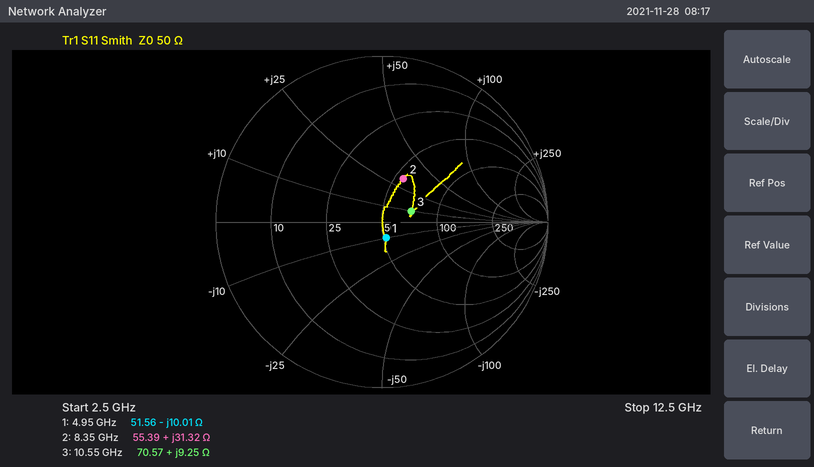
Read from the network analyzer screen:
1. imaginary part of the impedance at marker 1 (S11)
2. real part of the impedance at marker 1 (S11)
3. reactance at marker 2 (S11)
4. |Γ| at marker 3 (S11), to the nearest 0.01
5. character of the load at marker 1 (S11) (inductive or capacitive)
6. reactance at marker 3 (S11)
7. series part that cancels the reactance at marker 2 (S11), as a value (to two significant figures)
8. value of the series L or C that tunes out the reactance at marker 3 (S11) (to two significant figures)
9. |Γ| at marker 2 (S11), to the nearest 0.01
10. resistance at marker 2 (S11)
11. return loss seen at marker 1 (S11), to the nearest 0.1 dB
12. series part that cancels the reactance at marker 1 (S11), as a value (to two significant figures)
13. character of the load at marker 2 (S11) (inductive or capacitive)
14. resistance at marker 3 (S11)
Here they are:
-10.01 Ω
51.56 Ω
+31.32 Ω
0.19
capacitive
+9.25 Ω
610 fF
1.6 pF
0.29
55.39 Ω
20.1 dB
320 pH
inductive
70.57 Ω
